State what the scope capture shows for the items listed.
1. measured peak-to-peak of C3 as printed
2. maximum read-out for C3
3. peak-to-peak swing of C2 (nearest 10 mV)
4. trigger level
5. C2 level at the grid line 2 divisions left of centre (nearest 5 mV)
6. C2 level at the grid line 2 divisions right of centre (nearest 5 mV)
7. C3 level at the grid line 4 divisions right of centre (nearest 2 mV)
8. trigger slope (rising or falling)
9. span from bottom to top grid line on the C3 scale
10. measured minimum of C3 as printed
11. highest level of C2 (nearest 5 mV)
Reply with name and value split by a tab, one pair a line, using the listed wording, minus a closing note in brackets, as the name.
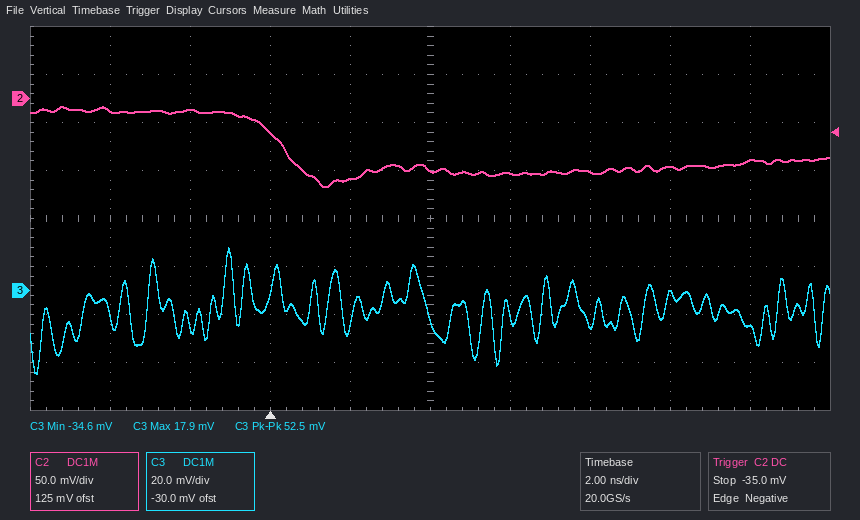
measured peak-to-peak of C3 as printed	52.5 mV
maximum read-out for C3	17.9 mV
peak-to-peak swing of C2	80 mV
trigger level	-35.0 mV
C2 level at the grid line 2 divisions left of centre	-35 mV
C2 level at the grid line 2 divisions right of centre	-75 mV
C3 level at the grid line 4 divisions right of centre	-16 mV
trigger slope	falling
span from bottom to top grid line on the C3 scale	160 mV
measured minimum of C3 as printed	-34.6 mV
highest level of C2	-10 mV
